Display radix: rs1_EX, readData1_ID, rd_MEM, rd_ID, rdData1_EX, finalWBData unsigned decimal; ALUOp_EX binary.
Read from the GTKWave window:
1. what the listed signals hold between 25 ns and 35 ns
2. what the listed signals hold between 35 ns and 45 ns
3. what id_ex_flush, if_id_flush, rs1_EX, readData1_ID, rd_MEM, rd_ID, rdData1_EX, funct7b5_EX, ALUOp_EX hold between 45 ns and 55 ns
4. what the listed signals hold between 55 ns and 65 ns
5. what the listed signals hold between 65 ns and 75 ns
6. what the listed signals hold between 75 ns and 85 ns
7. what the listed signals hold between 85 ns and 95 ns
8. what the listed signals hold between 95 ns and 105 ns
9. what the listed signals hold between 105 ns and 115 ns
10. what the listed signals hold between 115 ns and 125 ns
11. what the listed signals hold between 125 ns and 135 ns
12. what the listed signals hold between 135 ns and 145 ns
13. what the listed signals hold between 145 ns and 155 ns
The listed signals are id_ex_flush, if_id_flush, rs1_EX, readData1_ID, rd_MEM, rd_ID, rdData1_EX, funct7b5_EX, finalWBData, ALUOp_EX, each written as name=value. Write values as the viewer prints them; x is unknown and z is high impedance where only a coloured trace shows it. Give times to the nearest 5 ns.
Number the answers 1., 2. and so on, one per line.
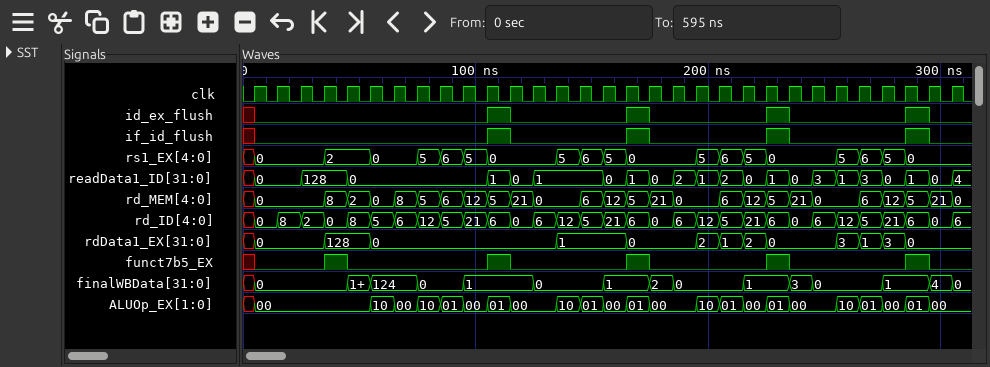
1. id_ex_flush=0, if_id_flush=0, rs1_EX=0, readData1_ID=128, rd_MEM=0, rd_ID=2, rdData1_EX=0, funct7b5_EX=0, finalWBData=0, ALUOp_EX=00
2. id_ex_flush=0, if_id_flush=0, rs1_EX=2, readData1_ID=128, rd_MEM=8, rd_ID=0, rdData1_EX=128, funct7b5_EX=1, finalWBData=0, ALUOp_EX=00
3. id_ex_flush=0, if_id_flush=0, rs1_EX=2, readData1_ID=0, rd_MEM=2, rd_ID=8, rdData1_EX=128, funct7b5_EX=0, ALUOp_EX=00
4. id_ex_flush=0, if_id_flush=0, rs1_EX=0, readData1_ID=0, rd_MEM=0, rd_ID=5, rdData1_EX=0, funct7b5_EX=0, finalWBData=124, ALUOp_EX=10
5. id_ex_flush=0, if_id_flush=0, rs1_EX=0, readData1_ID=0, rd_MEM=8, rd_ID=6, rdData1_EX=0, funct7b5_EX=0, finalWBData=124, ALUOp_EX=00
6. id_ex_flush=0, if_id_flush=0, rs1_EX=5, readData1_ID=0, rd_MEM=5, rd_ID=12, rdData1_EX=0, funct7b5_EX=0, finalWBData=0, ALUOp_EX=10
7. id_ex_flush=0, if_id_flush=0, rs1_EX=6, readData1_ID=0, rd_MEM=6, rd_ID=5, rdData1_EX=0, funct7b5_EX=0, finalWBData=0, ALUOp_EX=01
8. id_ex_flush=0, if_id_flush=0, rs1_EX=5, readData1_ID=0, rd_MEM=12, rd_ID=21, rdData1_EX=0, funct7b5_EX=0, finalWBData=1, ALUOp_EX=00
9. id_ex_flush=1, if_id_flush=1, rs1_EX=0, readData1_ID=1, rd_MEM=5, rd_ID=6, rdData1_EX=0, funct7b5_EX=1, finalWBData=1, ALUOp_EX=01
10. id_ex_flush=0, if_id_flush=0, rs1_EX=0, readData1_ID=0, rd_MEM=21, rd_ID=0, rdData1_EX=0, funct7b5_EX=0, finalWBData=1, ALUOp_EX=00
11. id_ex_flush=0, if_id_flush=0, rs1_EX=0, readData1_ID=1, rd_MEM=0, rd_ID=6, rdData1_EX=0, funct7b5_EX=0, finalWBData=0, ALUOp_EX=00
12. id_ex_flush=0, if_id_flush=0, rs1_EX=5, readData1_ID=1, rd_MEM=0, rd_ID=12, rdData1_EX=1, funct7b5_EX=0, finalWBData=0, ALUOp_EX=10
13. id_ex_flush=0, if_id_flush=0, rs1_EX=6, readData1_ID=1, rd_MEM=6, rd_ID=5, rdData1_EX=1, funct7b5_EX=0, finalWBData=0, ALUOp_EX=01
